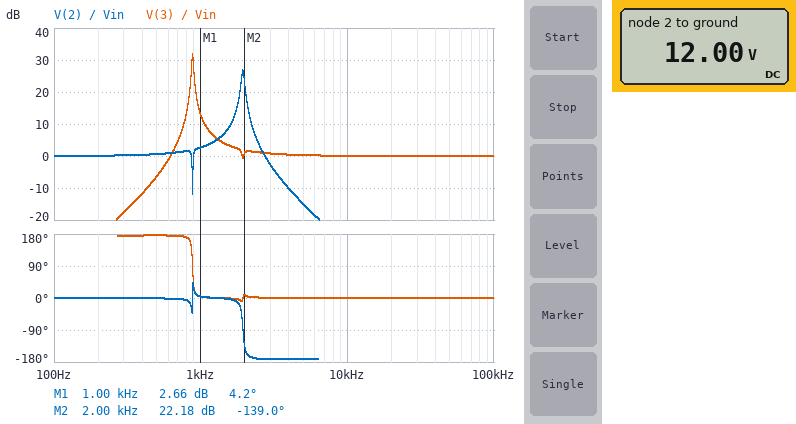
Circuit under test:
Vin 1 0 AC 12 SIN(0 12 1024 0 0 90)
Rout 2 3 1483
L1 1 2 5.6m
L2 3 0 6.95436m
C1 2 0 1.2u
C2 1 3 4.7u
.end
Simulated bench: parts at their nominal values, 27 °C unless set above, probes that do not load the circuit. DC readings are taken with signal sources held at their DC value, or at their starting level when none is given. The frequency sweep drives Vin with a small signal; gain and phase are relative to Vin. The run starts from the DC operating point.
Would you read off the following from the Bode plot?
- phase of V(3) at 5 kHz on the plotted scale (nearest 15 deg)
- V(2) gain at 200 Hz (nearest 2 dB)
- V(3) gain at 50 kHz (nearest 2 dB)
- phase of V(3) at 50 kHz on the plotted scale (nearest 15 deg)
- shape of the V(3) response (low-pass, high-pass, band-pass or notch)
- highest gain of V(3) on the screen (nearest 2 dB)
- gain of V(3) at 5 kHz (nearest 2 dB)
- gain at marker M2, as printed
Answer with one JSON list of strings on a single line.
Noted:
["0 deg", "0 dB", "0 dB", "0 deg", "high-pass", "32 dB", "0 dB", "22.18 dB"]
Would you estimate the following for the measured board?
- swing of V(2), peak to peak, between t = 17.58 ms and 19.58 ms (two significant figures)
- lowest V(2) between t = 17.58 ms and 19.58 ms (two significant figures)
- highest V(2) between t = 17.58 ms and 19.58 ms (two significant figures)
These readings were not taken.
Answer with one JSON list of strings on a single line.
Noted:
["34 V", "-17 V", "17 V"]
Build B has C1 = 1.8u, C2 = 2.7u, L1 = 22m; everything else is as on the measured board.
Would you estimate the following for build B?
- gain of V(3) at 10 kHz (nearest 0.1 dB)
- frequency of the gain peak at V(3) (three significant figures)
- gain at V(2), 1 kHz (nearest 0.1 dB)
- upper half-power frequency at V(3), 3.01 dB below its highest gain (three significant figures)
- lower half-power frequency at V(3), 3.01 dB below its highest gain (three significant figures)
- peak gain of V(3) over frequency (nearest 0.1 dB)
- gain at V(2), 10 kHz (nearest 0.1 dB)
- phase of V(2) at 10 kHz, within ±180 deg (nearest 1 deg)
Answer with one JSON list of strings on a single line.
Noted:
["0.1 dB", "1.16 kHz", "5.1 dB", "1.18 kHz", "1.14 kHz", "29.4 dB", "-41.1 dB", "-136 deg"]
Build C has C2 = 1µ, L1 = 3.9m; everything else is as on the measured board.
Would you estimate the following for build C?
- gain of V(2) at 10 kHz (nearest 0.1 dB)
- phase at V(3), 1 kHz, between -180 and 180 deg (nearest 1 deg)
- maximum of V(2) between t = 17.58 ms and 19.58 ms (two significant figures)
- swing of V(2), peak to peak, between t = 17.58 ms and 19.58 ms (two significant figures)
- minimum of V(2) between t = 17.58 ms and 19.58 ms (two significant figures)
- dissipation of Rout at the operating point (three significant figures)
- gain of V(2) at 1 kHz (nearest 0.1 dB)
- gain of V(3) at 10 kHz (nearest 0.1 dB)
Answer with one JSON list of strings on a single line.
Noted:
["-24.7 dB", "170 deg", "15 V", "30 V", "-15 V", "97.1 mW", "1.8 dB", "0.3 dB"]
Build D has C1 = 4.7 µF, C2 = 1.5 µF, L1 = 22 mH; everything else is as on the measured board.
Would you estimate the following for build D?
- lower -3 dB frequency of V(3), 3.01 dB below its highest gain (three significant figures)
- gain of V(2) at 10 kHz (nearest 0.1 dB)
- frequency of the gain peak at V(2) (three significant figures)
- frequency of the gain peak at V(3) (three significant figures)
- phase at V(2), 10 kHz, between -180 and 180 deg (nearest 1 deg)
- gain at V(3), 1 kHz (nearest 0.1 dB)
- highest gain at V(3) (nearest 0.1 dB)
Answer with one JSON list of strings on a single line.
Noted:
["1.52 kHz", "-49.4 dB", "495 Hz", "1.56 kHz", "-136 deg", "-3.1 dB", "26.8 dB"]
